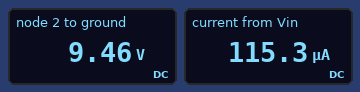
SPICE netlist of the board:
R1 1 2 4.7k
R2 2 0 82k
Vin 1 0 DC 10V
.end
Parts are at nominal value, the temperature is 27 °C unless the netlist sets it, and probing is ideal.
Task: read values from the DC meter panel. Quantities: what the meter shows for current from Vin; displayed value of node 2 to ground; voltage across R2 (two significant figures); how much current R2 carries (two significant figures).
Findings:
115.3 µA
9.46 V
9.5 V
120 µA
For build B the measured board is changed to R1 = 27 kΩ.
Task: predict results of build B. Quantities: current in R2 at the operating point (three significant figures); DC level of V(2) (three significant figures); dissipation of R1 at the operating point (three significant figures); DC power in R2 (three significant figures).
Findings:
91.7 µA
7.52 V
227 µW
690 µW
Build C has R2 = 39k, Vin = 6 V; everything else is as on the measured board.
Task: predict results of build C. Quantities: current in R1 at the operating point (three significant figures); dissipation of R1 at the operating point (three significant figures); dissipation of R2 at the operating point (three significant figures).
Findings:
137 µA
88.6 µW
735 µW
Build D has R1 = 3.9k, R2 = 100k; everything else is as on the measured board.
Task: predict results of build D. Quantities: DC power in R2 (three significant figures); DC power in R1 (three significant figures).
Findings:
926 µW
36.1 µW
